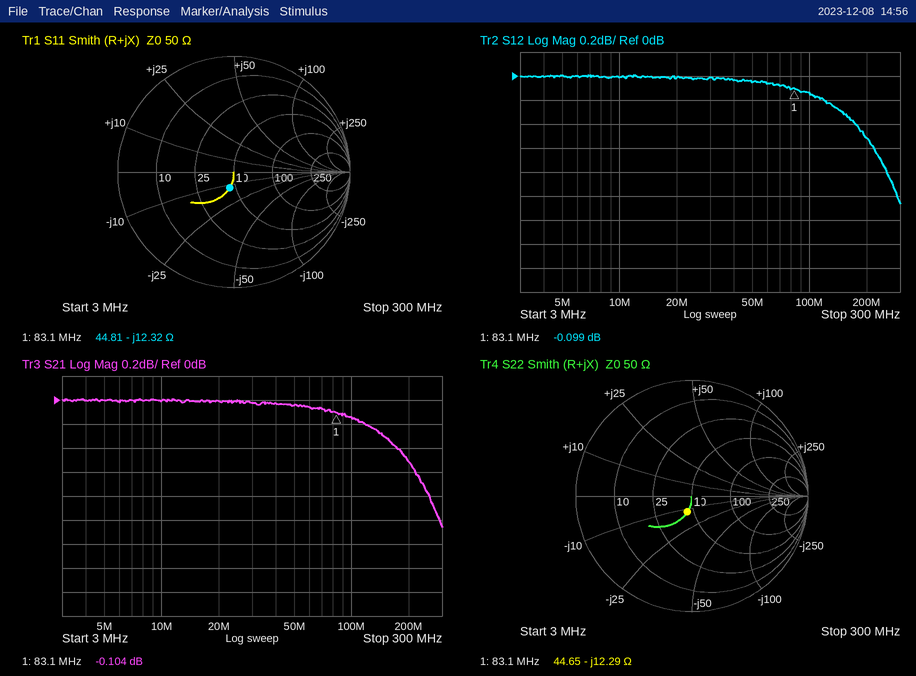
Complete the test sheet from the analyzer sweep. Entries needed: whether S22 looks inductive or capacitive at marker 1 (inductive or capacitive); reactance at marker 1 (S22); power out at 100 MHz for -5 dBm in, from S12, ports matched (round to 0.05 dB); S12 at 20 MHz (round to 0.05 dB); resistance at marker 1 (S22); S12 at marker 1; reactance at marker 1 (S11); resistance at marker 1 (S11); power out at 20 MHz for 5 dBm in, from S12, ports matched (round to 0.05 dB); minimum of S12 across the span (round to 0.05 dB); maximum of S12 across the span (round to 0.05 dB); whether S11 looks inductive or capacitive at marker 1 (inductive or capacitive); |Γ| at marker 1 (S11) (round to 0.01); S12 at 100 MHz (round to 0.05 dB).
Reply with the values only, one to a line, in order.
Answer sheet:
capacitive
-12.29 Ω
-5.15 dBm
0.00 dB
44.65 Ω
-0.099 dB
-12.32 Ω
44.81 Ω
5.00 dBm
-1.05 dB
0.00 dB
capacitive
0.14
-0.15 dB
